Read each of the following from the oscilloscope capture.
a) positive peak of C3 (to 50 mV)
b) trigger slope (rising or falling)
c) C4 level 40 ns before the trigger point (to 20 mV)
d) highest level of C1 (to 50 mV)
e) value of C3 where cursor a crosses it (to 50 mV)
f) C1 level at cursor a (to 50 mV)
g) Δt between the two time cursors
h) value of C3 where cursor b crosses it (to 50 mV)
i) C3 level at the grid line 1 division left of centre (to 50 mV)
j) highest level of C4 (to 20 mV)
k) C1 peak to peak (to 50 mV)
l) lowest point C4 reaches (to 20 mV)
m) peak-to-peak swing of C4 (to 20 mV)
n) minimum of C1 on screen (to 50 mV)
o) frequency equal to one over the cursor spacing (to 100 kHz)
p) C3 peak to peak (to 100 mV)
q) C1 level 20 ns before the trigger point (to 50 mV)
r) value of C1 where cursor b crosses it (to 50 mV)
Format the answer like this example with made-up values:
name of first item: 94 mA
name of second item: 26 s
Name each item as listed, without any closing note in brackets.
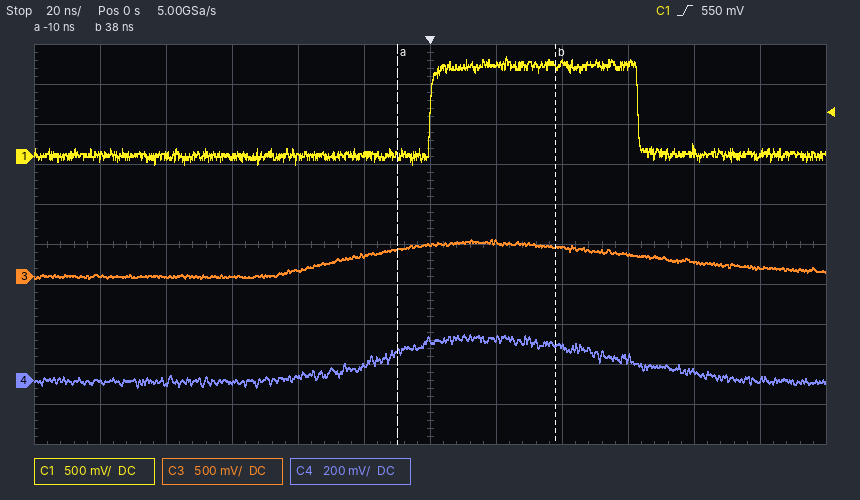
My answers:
positive peak of C3: 450 mV
trigger slope: rising
C4 level 40 ns before the trigger point: 20 mV
highest level of C1: 1.25 V
value of C3 where cursor a crosses it: 350 mV
C1 level at cursor a: 0 mV
Δt between the two time cursors: 48 ns
value of C3 where cursor b crosses it: 350 mV
C3 level at the grid line 1 division left of centre: 250 mV
highest level of C4: 220 mV
C1 peak to peak: 1.35 V
lowest point C4 reaches: -40 mV
peak-to-peak swing of C4: 260 mV
minimum of C1 on screen: -100 mV
frequency equal to one over the cursor spacing: 20.8 MHz
C3 peak to peak: 500 mV
C1 level 20 ns before the trigger point: 0 mV
value of C1 where cursor b crosses it: 1.15 V
